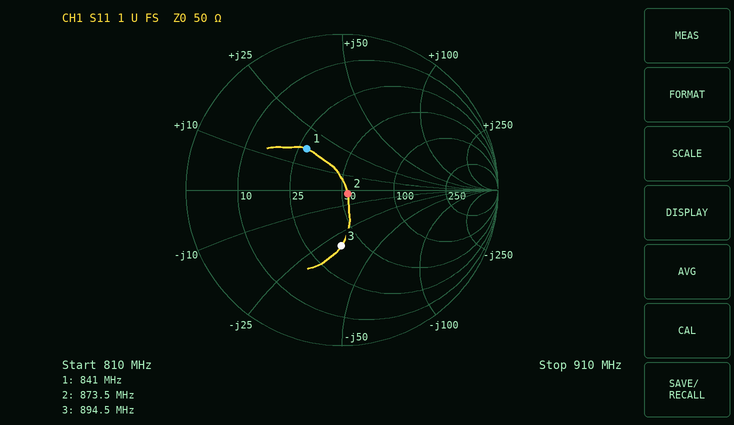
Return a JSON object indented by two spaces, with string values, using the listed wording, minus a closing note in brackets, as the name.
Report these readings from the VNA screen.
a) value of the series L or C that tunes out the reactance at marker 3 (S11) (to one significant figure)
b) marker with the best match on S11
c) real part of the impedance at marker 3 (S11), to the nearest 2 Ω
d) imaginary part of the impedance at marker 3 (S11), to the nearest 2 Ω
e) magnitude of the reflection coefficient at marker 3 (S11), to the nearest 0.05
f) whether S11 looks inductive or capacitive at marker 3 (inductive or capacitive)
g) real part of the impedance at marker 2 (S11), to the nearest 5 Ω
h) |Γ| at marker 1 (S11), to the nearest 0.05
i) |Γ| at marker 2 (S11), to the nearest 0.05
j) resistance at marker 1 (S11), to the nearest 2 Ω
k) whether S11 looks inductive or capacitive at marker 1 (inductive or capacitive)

{
  "value of the series L or C that tunes out the reactance at marker 3 (S11)": "6 nH",
  "marker with the best match on S11": "marker 2",
  "real part of the impedance at marker 3 (S11), to the nearest 2 Ω": "38 Ω",
  "imaginary part of the impedance at marker 3 (S11), to the nearest 2 Ω": "-32 Ω",
  "magnitude of the reflection coefficient at marker 3 (S11), to the nearest 0.05": "0.35",
  "whether S11 looks inductive or capacitive at marker 3": "capacitive",
  "real part of the impedance at marker 2 (S11), to the nearest 5 Ω": "55 Ω",
  "|Γ| at marker 1 (S11), to the nearest 0.05": "0.35",
  "|Γ| at marker 2 (S11), to the nearest 0.05": "0.05",
  "resistance at marker 1 (S11), to the nearest 2 Ω": "28 Ω",
  "whether S11 looks inductive or capacitive at marker 1": "inductive"
}
